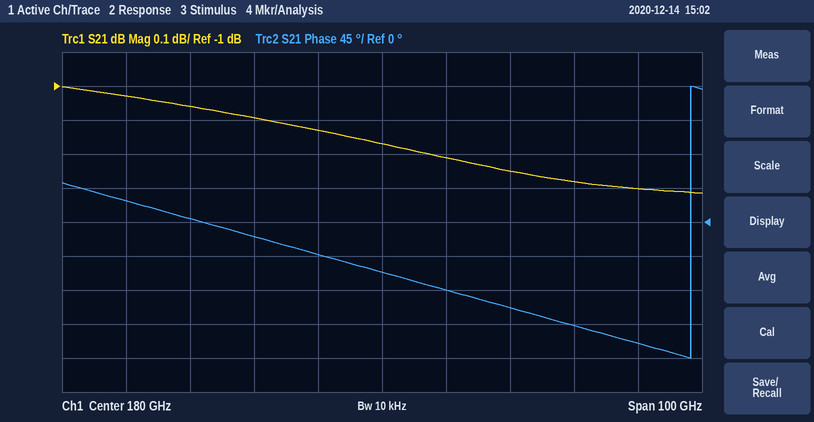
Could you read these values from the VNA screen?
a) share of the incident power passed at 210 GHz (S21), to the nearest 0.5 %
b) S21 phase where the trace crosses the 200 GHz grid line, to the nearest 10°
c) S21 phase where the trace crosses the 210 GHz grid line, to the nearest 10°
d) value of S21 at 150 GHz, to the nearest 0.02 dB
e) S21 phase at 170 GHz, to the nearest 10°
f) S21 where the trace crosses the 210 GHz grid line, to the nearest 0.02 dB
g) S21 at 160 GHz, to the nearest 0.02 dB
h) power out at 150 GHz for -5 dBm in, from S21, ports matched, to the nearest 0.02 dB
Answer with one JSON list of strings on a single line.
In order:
["74.5 %", "-110°", "-140°", "-1.06 dB", "-40°", "-1.28 dB", "-1.10 dB", "-6.06 dBm"]
